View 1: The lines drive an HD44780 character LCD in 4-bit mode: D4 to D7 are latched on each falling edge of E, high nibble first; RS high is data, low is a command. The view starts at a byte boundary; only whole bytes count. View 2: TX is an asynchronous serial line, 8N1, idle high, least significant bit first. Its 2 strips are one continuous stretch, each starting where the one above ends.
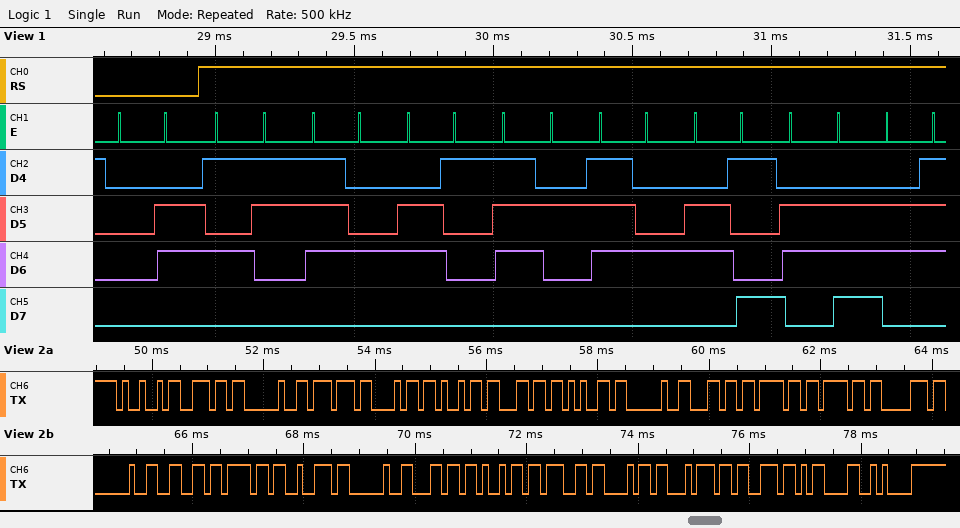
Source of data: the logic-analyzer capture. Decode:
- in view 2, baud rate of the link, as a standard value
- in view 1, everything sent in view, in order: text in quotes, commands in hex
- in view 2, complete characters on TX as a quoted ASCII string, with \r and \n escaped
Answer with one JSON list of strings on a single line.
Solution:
["9600 baud", "0x06 \"Starting\"", "\"In while loop for lights\\r\\n\""]
